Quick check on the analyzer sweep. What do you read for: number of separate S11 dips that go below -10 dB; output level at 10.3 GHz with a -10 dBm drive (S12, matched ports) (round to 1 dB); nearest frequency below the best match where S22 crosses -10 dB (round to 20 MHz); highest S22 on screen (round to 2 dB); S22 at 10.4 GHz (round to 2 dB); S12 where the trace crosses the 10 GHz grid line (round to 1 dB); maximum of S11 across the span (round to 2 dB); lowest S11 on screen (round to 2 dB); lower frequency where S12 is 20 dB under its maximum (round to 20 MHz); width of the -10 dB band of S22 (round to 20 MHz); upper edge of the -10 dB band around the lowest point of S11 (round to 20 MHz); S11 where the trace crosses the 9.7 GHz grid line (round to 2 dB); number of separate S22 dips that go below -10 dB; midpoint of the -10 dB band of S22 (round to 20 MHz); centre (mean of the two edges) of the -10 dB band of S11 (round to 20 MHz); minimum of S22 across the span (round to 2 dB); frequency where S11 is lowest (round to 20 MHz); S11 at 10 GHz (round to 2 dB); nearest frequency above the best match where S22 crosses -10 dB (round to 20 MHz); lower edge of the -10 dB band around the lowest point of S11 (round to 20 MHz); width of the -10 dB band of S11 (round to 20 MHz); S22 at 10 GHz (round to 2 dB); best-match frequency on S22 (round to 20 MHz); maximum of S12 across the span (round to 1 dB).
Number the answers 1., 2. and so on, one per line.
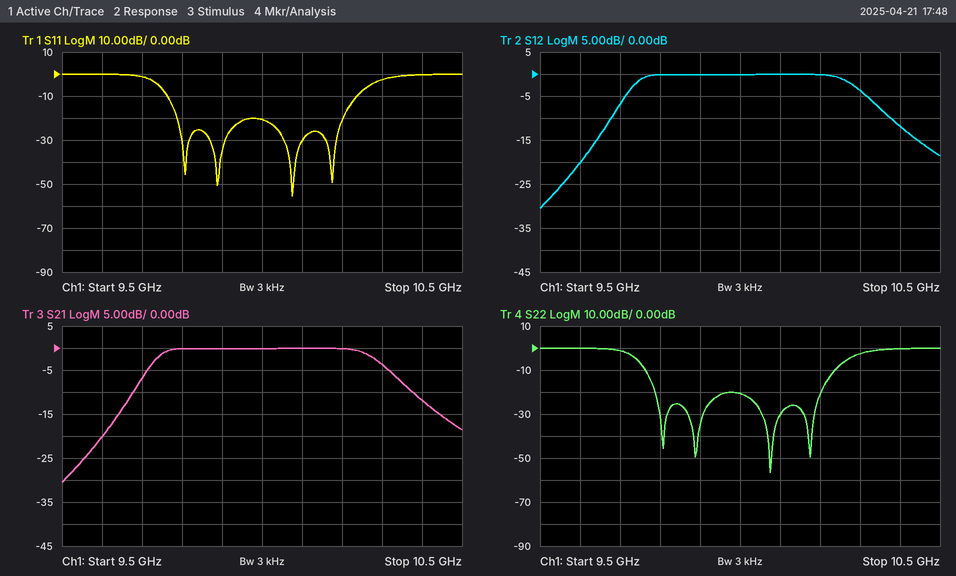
1. 4
2. -14 dBm
3. 9.76 GHz
4. 0 dB
5. 0 dB
6. 0 dB
7. 0 dB
8. -56 dB
9. 9.60 GHz
10. 480 MHz
11. 10.24 GHz
12. -2 dB
13. 4
14. 10.00 GHz
15. 10.00 GHz
16. -56 dB
17. 10.08 GHz
18. -20 dB
19. 10.24 GHz
20. 9.76 GHz
21. 480 MHz
22. -20 dB
23. 10.08 GHz
24. 0 dB
